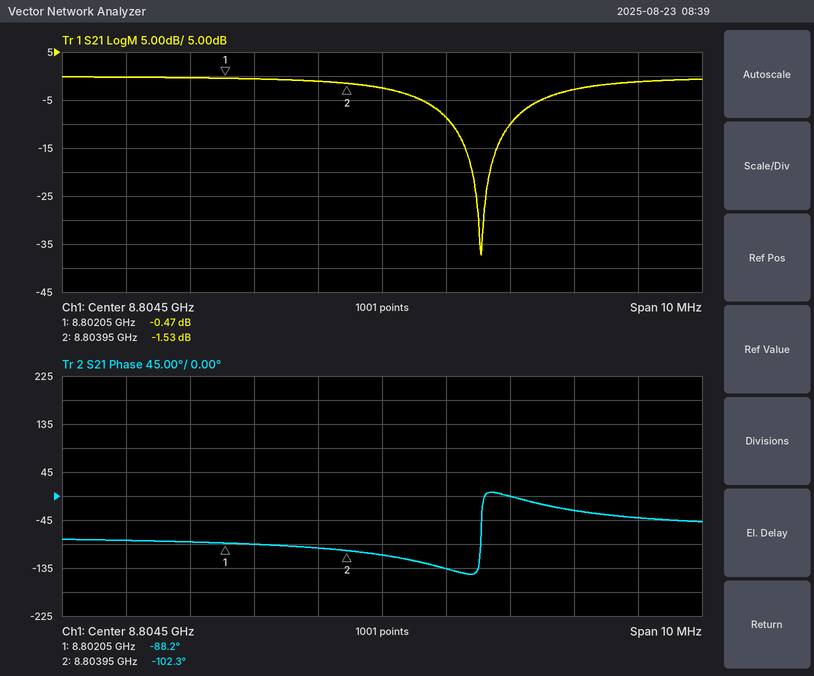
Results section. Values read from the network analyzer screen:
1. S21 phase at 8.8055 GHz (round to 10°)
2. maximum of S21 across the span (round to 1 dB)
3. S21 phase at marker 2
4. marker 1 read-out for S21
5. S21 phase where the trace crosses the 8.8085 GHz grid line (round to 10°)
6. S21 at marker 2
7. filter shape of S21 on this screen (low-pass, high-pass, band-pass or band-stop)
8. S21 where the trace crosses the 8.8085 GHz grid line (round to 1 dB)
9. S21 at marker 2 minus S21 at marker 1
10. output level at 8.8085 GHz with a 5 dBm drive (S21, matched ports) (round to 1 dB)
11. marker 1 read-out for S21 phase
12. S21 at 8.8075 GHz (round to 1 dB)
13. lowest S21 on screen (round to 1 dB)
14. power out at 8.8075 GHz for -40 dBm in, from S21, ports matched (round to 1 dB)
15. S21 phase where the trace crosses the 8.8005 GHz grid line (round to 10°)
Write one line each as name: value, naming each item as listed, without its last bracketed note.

S21 phase at 8.8055 GHz: -140°
maximum of S21 across the span: 0 dB
S21 phase at marker 2: -102.3°
marker 1 read-out for S21: -0.47 dB
S21 phase where the trace crosses the 8.8085 GHz grid line: -40°
S21 at marker 2: -1.53 dB
filter shape of S21 on this screen: band-stop
S21 where the trace crosses the 8.8085 GHz grid line: -1 dB
S21 at marker 2 minus S21 at marker 1: -1.06 dB
output level at 8.8085 GHz with a 5 dBm drive (S21, matched ports): 4 dBm
marker 1 read-out for S21 phase: -88.2°
S21 at 8.8075 GHz: -3 dB
lowest S21 on screen: -37 dB
power out at 8.8075 GHz for -40 dBm in, from S21, ports matched: -43 dBm
S21 phase where the trace crosses the 8.8005 GHz grid line: -80°
